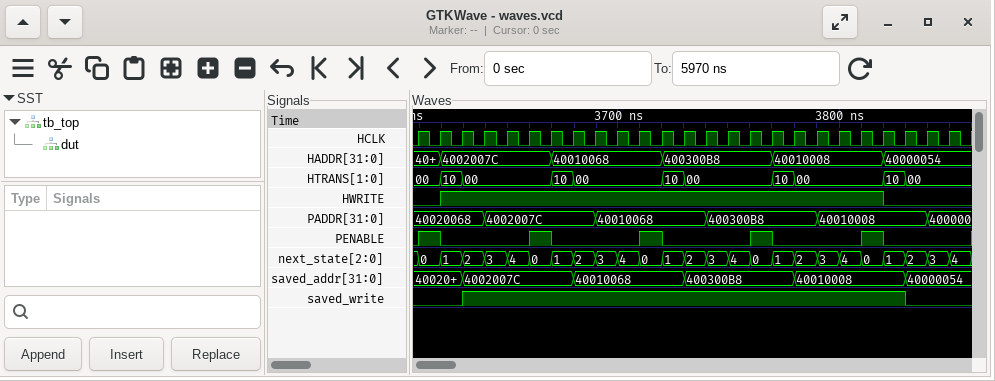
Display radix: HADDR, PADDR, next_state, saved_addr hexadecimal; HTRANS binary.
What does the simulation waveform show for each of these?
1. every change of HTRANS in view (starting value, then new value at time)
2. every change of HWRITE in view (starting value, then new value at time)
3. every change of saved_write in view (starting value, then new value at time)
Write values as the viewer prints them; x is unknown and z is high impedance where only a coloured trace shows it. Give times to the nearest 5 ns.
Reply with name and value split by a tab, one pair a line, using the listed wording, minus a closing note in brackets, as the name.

every change of HTRANS in view	00, 10 at 3620 ns, 00 at 3630 ns, 10 at 3670 ns, 00 at 3680 ns, 10 at 3720 ns, 00 at 3730 ns, 10 at 3770 ns, 00 at 3780 ns, 10 at 3820 ns, 00 at 3830 ns
every change of HWRITE in view	0, 1 at 3620 ns, 0 at 3820 ns
every change of saved_write in view	0, 1 at 3630 ns, 0 at 3830 ns
